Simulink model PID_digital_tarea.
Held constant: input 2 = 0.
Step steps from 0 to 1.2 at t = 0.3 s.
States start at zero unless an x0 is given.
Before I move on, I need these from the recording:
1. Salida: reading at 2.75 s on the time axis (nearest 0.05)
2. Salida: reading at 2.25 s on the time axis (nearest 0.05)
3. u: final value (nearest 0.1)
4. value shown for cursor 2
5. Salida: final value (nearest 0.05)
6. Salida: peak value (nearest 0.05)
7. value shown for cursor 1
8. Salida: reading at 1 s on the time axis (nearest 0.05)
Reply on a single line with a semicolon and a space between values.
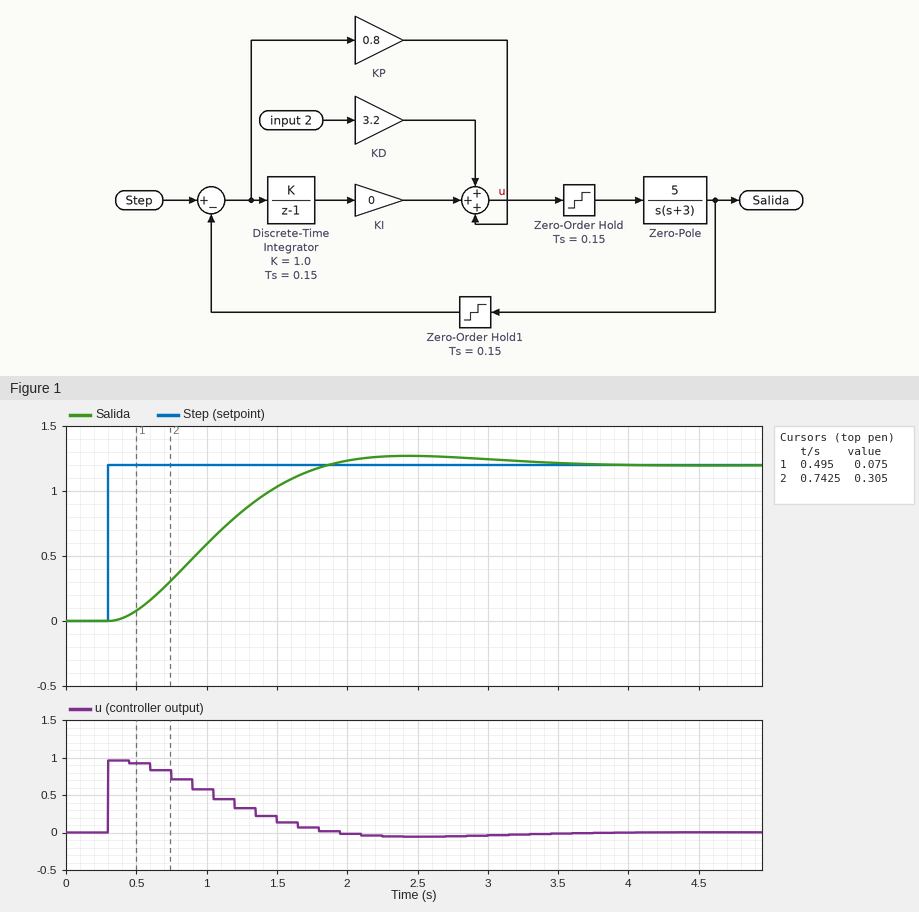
1.25; 1.25; 0.0; 0.305; 1.20; 1.25; 0.075; 0.60
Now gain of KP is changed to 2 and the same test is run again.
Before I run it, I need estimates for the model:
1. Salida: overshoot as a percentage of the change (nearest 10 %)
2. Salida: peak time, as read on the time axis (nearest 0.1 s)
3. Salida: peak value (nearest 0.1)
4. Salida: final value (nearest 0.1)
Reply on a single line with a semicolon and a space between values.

30 %; 1.4 s; 1.6; 1.2
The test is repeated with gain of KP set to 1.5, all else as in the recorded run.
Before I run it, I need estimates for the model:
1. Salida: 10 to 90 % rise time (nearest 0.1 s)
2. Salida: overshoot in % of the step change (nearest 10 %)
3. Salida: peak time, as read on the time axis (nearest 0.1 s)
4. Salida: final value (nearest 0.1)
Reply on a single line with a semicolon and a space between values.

0.6 s; 20 %; 1.6 s; 1.2
